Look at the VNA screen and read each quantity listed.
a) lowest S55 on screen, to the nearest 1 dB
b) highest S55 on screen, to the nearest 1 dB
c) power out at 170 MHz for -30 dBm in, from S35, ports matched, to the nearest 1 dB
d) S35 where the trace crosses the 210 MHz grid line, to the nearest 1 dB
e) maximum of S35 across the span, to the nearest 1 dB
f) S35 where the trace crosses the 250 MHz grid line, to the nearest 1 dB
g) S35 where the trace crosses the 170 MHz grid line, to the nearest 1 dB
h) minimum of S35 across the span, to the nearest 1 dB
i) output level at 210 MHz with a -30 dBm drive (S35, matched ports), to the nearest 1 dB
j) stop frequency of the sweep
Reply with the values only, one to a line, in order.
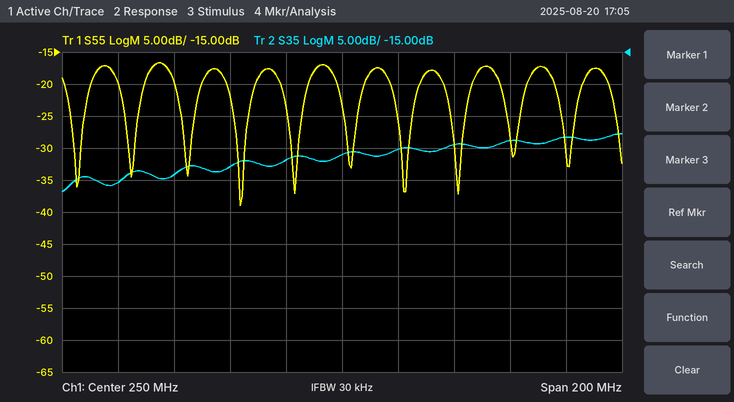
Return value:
-39 dB
-17 dB
-65 dBm
-33 dB
-28 dB
-31 dB
-35 dB
-37 dB
-63 dBm
350 MHz
